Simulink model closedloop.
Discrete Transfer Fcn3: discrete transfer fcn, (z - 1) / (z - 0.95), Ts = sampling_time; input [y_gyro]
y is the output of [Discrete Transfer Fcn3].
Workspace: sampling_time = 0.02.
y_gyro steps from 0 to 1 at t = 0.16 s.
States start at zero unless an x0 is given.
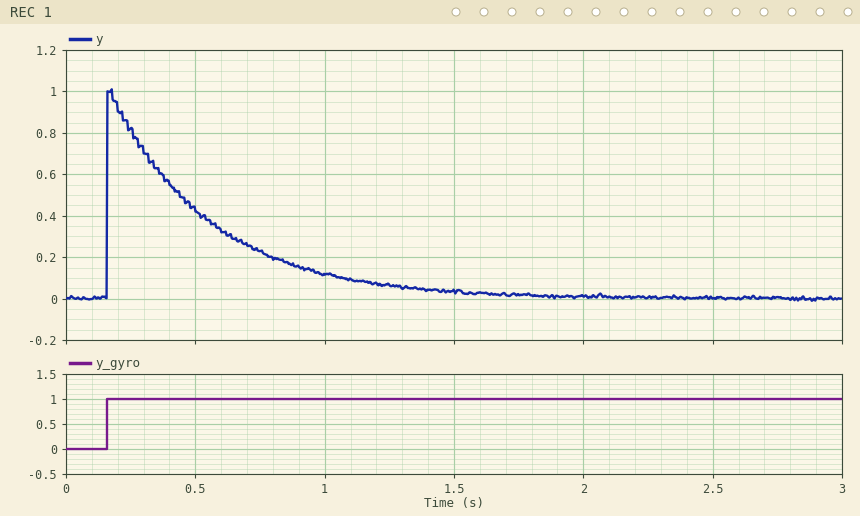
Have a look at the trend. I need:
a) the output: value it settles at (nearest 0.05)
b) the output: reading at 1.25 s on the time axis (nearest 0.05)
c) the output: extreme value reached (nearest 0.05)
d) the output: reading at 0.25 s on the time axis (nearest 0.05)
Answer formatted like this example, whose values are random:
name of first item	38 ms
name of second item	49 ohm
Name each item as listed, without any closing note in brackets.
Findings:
the output: value it settles at	0.00
the output: reading at 1.25 s on the time axis	0.05
the output: extreme value reached	1.00
the output: reading at 0.25 s on the time axis	0.80
